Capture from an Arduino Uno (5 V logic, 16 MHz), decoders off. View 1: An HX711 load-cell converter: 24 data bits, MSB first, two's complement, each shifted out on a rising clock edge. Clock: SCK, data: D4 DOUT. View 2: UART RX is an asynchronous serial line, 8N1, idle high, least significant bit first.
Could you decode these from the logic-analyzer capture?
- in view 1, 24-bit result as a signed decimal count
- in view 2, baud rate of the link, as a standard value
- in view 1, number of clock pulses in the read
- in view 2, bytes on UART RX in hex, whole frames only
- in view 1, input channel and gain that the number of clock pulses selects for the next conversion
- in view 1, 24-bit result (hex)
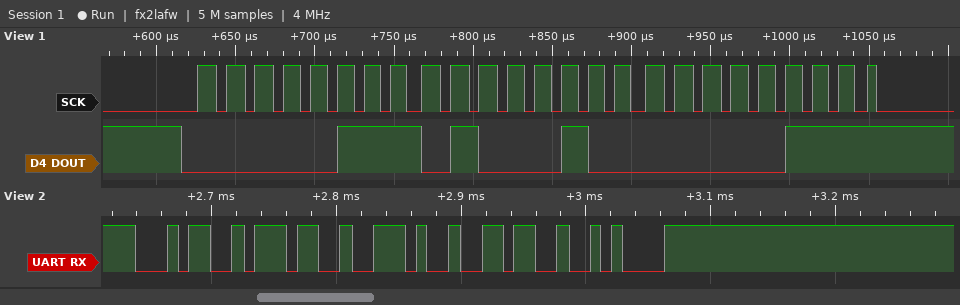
476167
115200 baud
25
0x34 0x37 0x2E 0x36 0x0A
channel A, gain 128
0x074407
